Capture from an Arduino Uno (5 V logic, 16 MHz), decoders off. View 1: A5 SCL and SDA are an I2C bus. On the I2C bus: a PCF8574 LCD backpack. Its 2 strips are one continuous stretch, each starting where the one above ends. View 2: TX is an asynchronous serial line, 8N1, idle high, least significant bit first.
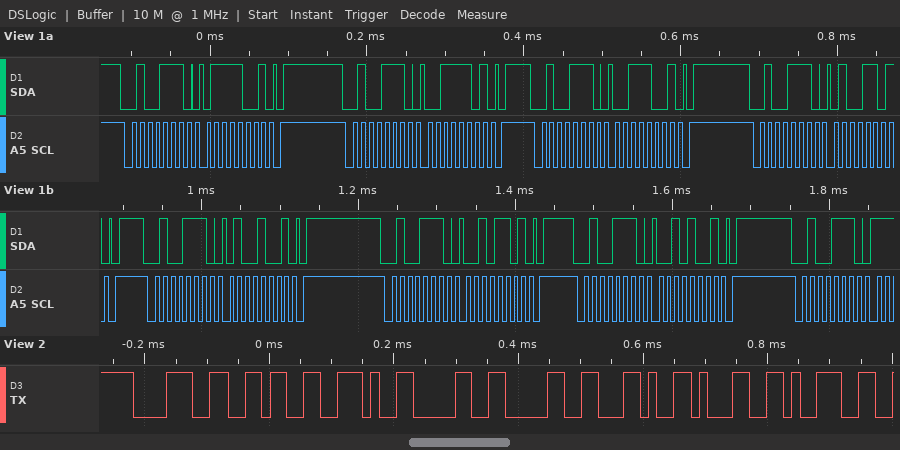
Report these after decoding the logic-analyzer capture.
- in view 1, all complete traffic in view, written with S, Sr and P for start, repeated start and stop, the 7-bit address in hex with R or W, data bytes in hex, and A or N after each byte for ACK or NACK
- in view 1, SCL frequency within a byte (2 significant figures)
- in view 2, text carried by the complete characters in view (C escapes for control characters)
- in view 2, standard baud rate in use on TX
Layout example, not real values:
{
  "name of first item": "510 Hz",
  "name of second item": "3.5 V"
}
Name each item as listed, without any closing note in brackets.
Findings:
{
  "in view 1, all complete traffic in view, written with S, Sr and P for start, repeated start and stop, the 7-bit address in hex with R or W, data bytes in hex, and A or N after each byte for ACK or NACK": "S 27W A 79 A P S 27W A 3D A P S 27W A 39 A P S 27W A 4D A P S 27W A 49 A P S 27W A 2D A P S 27W A 29 A P S 27W A",
  "in view 1, SCL frequency within a byte": "100 kHz",
  "in view 2, text carried by the complete characters in view": "\"86.00,19\"",
  "in view 2, standard baud rate in use on TX": "74880 baud"
}
